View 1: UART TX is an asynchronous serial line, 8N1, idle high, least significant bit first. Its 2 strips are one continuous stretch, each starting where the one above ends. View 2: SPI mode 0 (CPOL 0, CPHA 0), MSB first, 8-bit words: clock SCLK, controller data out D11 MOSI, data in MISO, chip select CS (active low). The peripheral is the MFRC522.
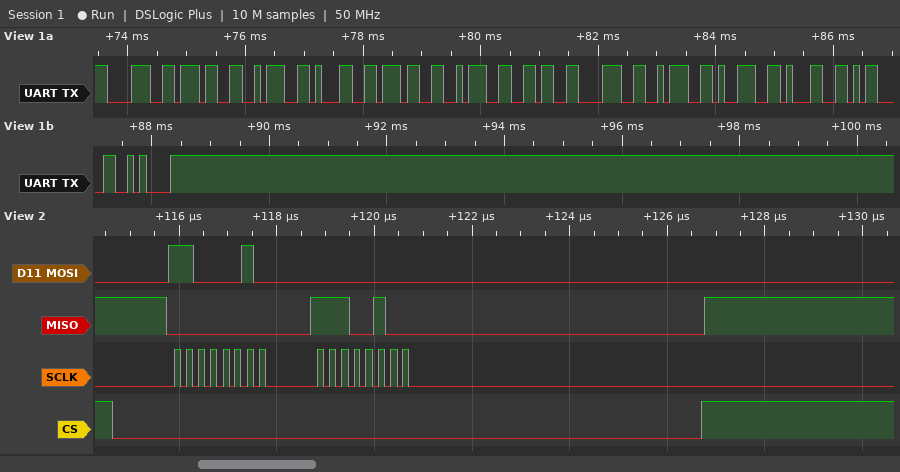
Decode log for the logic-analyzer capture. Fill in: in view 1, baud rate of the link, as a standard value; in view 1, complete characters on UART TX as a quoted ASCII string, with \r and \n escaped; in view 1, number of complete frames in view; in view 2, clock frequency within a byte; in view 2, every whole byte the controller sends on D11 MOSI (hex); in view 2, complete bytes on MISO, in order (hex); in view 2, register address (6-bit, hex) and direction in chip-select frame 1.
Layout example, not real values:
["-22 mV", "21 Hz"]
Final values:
["9600 baud", "\"87:17:68:91\\r\\n\"", "13", "4 MHz", "C2 00", "00 E4", "0x21 read"]
